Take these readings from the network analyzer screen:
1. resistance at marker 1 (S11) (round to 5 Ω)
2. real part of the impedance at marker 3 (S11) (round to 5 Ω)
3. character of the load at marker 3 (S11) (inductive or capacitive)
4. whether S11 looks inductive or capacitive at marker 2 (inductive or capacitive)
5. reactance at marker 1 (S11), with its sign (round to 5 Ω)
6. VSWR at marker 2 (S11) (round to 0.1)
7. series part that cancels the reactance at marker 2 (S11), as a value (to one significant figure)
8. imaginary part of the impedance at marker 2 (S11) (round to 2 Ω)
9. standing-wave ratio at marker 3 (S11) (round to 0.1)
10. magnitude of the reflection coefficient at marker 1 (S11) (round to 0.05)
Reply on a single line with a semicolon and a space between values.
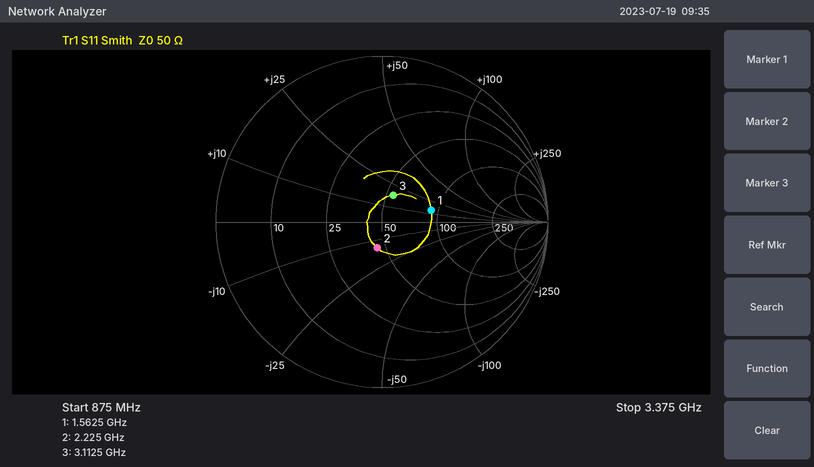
90 Ω; 55 Ω; inductive; capacitive; +15 Ω; 1.4; 1 nH; -14 Ω; 1.4; 0.30
